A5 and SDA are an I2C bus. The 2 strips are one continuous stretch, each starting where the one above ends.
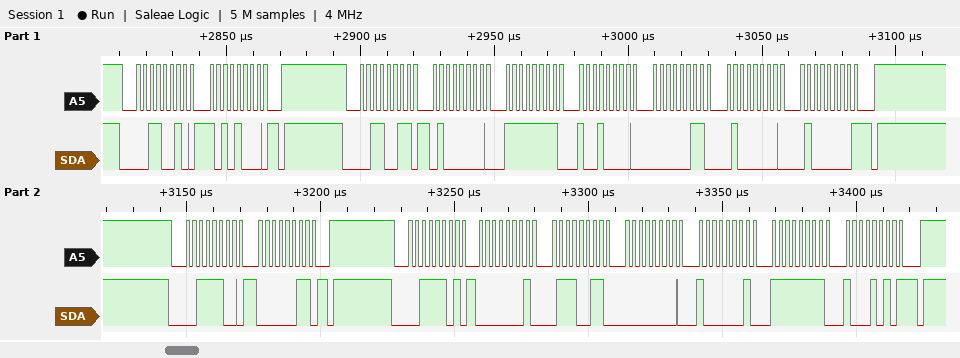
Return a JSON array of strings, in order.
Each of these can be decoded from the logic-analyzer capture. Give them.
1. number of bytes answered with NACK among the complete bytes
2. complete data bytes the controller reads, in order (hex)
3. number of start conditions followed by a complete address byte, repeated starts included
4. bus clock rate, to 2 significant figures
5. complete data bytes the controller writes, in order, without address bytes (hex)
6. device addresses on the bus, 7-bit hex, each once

["2", "40 FF 90 03 40 40 01 73 00 81 FF 8A", "4", "400 kHz", "A8 03", "0x19 0x1E"]
